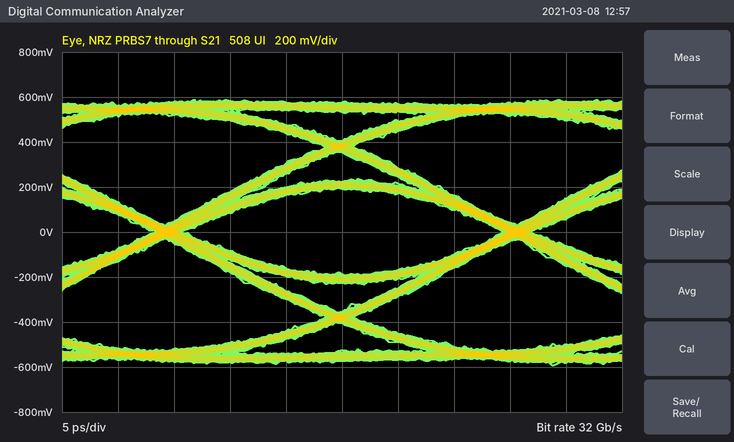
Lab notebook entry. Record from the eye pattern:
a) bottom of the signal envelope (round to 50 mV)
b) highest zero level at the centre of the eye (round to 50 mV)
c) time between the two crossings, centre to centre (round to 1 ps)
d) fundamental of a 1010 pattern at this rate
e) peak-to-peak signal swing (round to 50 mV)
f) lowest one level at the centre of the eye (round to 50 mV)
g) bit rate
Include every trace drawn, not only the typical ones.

-600 mV
-200 mV
31 ps
16 GHz
1.20 V
200 mV
32 Gb/s
